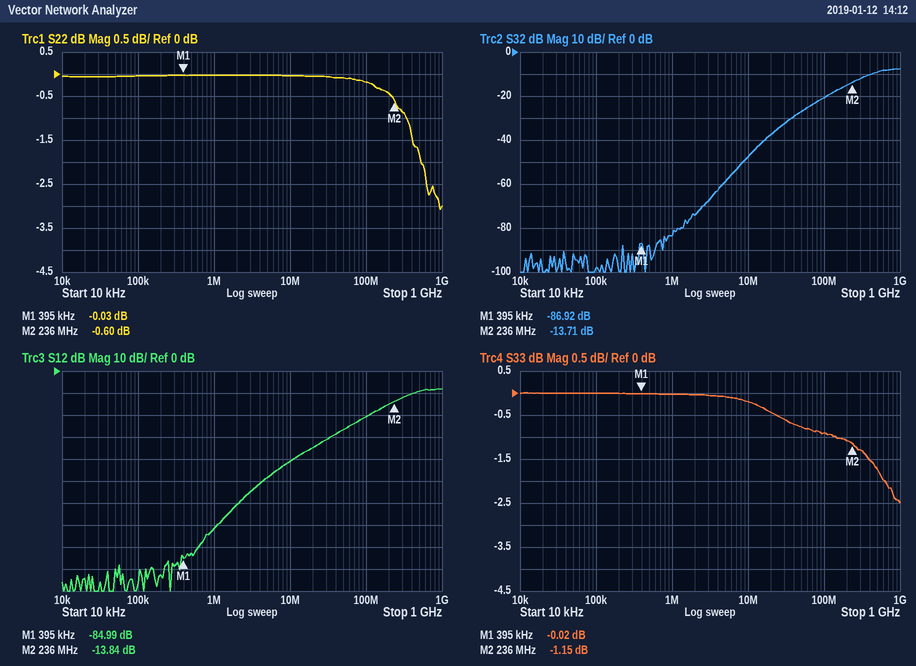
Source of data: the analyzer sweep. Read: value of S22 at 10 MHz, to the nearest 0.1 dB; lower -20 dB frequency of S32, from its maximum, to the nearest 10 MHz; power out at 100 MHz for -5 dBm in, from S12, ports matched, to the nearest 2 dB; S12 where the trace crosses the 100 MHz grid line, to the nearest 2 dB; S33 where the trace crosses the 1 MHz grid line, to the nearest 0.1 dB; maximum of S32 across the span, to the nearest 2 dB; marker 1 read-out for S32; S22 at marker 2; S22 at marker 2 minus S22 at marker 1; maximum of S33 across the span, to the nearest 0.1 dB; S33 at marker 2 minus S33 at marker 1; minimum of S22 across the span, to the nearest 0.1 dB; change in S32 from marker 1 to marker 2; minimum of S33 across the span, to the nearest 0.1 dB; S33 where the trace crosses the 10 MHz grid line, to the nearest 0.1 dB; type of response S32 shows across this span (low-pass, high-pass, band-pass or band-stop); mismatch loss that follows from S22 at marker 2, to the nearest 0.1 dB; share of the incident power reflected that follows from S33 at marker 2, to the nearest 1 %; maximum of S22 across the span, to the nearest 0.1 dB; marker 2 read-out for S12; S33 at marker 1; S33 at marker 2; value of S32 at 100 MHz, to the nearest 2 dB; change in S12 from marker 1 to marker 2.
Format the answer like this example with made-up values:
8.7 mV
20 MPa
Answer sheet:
0.0 dB
50 MHz
-26 dBm
-20 dB
0.0 dB
-8 dB
-86.92 dB
-0.60 dB
-0.57 dB
0.0 dB
-1.13 dB
-3.1 dB
73.21 dB
-2.5 dB
-0.2 dB
high-pass
8.9 dB
77 %
0.0 dB
-13.84 dB
-0.02 dB
-1.15 dB
-20 dB
71.15 dB
